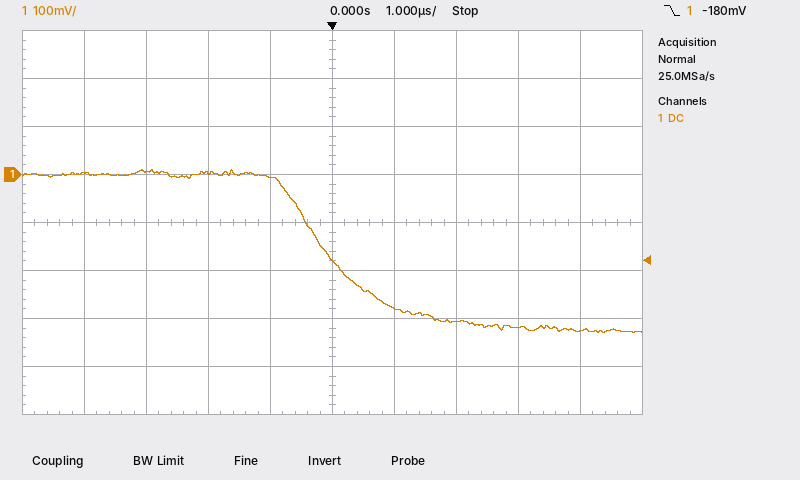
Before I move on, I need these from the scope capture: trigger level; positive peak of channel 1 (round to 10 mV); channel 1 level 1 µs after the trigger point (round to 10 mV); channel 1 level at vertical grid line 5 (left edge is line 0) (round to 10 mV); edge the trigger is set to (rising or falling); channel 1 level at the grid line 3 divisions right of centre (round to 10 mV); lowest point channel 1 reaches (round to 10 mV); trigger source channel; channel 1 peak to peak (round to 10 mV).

-180 mV
10 mV
-280 mV
-180 mV
falling
-320 mV
-330 mV
channel 1
340 mV
